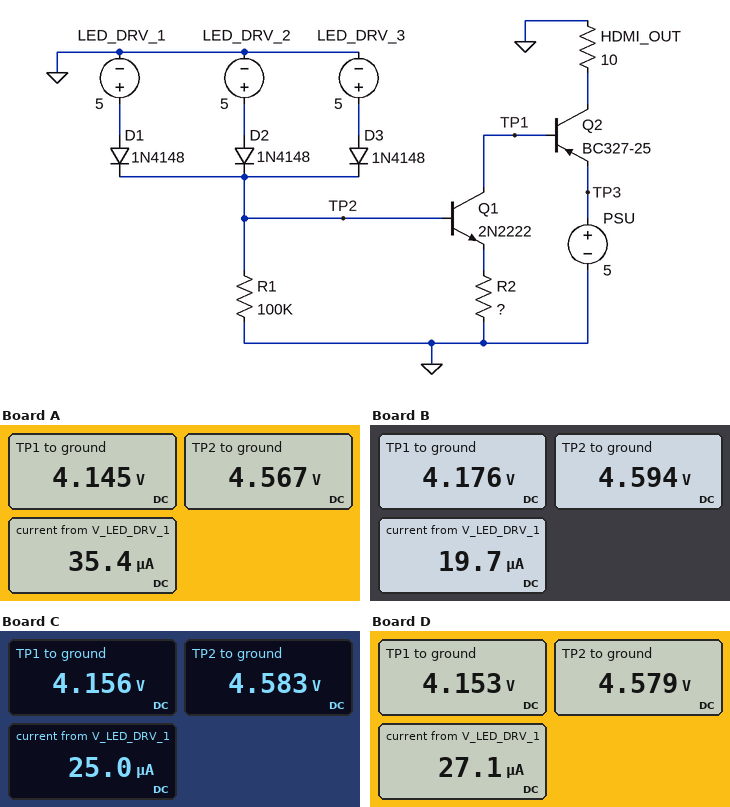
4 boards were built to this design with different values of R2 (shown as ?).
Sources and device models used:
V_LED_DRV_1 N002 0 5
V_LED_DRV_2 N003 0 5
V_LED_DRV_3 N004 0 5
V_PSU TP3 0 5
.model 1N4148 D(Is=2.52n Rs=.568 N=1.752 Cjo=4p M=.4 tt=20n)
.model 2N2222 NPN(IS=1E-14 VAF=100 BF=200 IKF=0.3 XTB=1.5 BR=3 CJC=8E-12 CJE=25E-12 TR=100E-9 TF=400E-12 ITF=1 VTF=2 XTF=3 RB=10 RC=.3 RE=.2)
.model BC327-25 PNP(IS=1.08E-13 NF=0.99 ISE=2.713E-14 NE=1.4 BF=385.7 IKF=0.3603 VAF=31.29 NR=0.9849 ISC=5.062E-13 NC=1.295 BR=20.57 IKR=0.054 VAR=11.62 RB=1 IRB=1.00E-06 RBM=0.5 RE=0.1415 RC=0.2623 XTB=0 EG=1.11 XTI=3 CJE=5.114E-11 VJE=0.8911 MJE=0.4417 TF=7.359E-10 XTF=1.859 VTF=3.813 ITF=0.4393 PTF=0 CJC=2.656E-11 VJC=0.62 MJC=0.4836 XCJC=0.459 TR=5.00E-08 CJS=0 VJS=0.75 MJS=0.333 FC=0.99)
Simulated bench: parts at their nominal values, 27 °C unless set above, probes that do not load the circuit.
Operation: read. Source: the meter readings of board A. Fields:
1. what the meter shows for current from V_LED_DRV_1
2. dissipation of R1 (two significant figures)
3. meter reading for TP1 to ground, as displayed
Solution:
35.4 µA
210 µW
4.145 V
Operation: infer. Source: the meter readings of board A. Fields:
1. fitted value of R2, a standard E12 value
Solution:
330 Ω
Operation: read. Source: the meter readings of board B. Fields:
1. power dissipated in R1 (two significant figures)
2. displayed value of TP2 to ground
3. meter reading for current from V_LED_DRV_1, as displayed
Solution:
210 µW
4.594 V
19.7 µA
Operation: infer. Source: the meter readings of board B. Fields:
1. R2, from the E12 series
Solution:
1.5 kΩ
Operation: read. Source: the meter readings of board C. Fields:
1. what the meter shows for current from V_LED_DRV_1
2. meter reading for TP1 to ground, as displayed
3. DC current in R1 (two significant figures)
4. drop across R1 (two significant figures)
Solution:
25.0 µA
4.156 V
46 µA
4.6 V
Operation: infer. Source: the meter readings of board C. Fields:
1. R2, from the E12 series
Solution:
680 Ω
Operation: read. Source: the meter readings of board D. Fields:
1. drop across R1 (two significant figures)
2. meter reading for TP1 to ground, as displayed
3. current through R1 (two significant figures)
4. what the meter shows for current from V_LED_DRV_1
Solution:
4.6 V
4.153 V
46 µA
27.1 µA
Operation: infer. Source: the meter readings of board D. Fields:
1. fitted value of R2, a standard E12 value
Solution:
560 Ω
